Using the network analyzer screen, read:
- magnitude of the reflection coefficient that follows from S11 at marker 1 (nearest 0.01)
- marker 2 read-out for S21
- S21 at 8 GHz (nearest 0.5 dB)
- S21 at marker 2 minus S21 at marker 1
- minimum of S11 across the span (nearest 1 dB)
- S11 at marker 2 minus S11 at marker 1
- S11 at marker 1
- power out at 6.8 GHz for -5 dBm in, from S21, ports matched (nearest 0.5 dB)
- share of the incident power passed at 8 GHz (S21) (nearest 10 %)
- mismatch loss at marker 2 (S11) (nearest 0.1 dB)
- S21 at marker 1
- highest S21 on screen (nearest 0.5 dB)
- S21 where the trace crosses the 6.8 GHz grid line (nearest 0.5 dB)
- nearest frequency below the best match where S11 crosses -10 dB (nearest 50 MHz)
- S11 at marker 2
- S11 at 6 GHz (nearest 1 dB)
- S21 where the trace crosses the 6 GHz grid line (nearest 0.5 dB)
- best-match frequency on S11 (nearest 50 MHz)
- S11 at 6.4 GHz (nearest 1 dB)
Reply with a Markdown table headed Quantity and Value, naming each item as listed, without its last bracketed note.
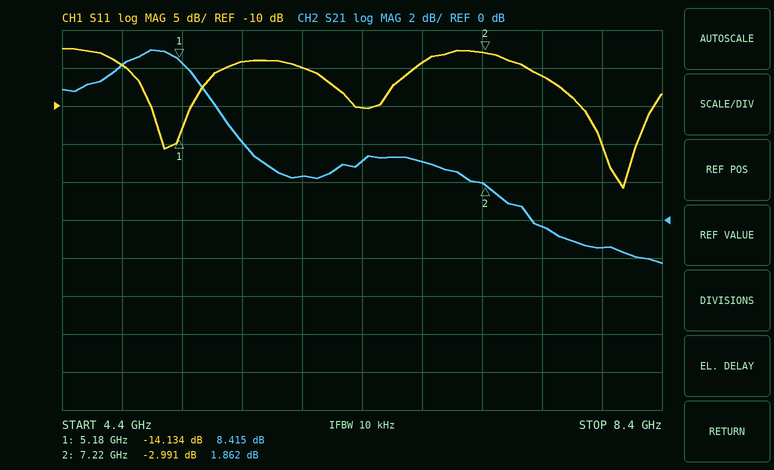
| Quantity | Value |
|---|---|
| magnitude of the reflection coefficient that follows from S11 at marker 1 | 0.20 |
| marker 2 read-out for S21 | 1.862 dB |
| S21 at 8 GHz | -1.5 dB |
| S21 at marker 2 minus S21 at marker 1 | -6.553 dB |
| minimum of S11 across the span | -21 dB |
| S11 at marker 2 minus S11 at marker 1 | 11.143 dB |
| S11 at marker 1 | -14.134 dB |
| power out at 6.8 GHz for -5 dBm in, from S21, ports matched | -2.0 dBm |
| share of the incident power passed at 8 GHz (S21) | 70 % |
| mismatch loss at marker 2 (S11) | 3.0 dB |
| S21 at marker 1 | 8.415 dB |
| highest S21 on screen | 9.0 dB |
| S21 where the trace crosses the 6.8 GHz grid line | 3.0 dB |
| nearest frequency below the best match where S11 crosses -10 dB | 7.85 GHz |
| S11 at marker 2 | -2.991 dB |
| S11 at 6 GHz | -5 dB |
| S21 where the trace crosses the 6 GHz grid line | 2.5 dB |
| best-match frequency on S11 | 8.15 GHz |
| S11 at 6.4 GHz | -10 dB |
